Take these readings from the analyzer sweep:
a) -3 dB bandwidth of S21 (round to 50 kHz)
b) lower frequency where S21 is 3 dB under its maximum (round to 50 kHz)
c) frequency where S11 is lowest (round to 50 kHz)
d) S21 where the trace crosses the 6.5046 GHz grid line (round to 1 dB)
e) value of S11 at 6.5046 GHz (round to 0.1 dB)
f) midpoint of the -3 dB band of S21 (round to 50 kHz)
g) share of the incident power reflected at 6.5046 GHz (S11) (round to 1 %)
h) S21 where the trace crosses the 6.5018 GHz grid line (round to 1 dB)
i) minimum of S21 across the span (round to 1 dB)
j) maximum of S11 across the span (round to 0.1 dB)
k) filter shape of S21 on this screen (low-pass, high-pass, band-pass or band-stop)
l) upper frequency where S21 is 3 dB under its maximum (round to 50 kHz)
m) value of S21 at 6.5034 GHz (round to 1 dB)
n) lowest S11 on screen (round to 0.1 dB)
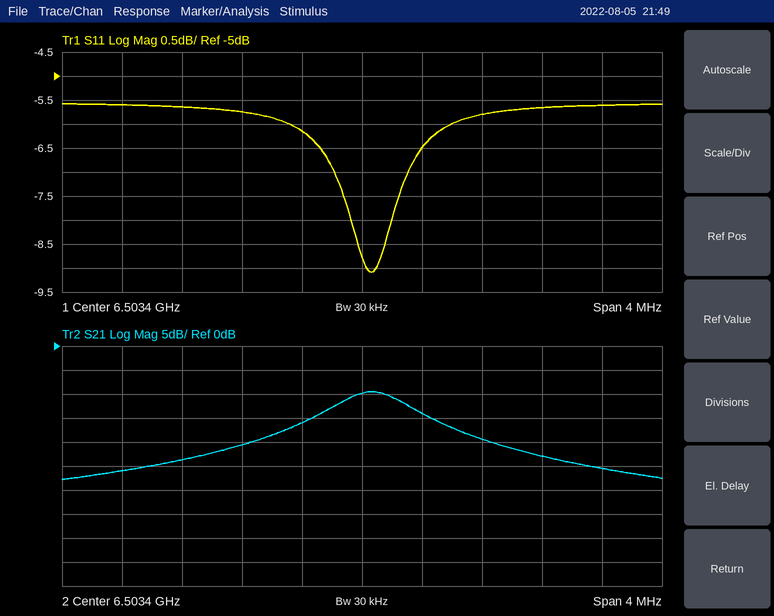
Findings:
500 kHz
6.50320 GHz
6.50345 GHz
-23 dB
-5.7 dB
6.50345 GHz
27 %
-26 dB
-28 dB
-5.6 dB
band-pass
6.50370 GHz
-10 dB
-9.1 dB
